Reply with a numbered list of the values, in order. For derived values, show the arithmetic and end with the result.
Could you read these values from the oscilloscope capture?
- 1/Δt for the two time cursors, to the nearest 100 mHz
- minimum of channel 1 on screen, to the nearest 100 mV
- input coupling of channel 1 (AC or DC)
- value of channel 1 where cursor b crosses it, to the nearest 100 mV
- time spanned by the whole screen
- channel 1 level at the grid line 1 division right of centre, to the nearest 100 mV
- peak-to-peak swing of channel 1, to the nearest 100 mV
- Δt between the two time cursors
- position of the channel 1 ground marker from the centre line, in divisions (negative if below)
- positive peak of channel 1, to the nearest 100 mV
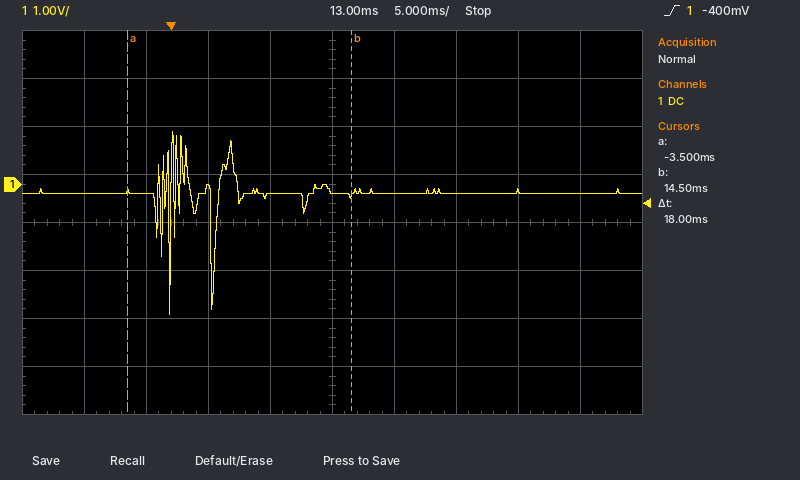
1. 1 / 18 ms ≈ 55.6 Hz
2. -2.7 V
3. DC
4. -200 mV
5. 50 ms
6. -200 mV
7. 1.1 V − (-2.7 V) = 3.8 V
8. 18 ms
9. +0.8 div
10. 1.1 V
